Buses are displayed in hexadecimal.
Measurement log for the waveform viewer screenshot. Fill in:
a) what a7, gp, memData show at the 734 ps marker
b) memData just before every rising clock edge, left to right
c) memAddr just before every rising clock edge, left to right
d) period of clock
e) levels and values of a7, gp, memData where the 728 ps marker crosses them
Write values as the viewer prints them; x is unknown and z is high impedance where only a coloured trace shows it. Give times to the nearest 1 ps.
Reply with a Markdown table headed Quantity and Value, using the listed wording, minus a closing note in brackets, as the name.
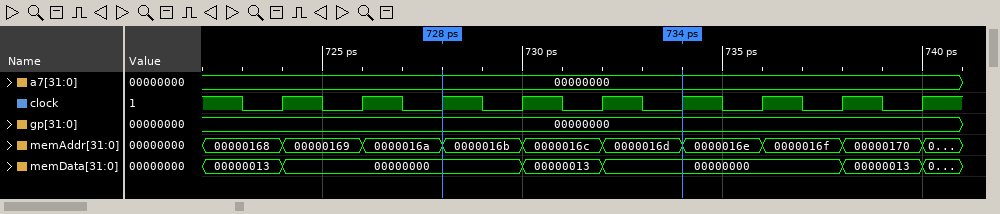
| Quantity | Value |
|---|---|
| what a7, gp, memData show at the 734 ps marker | a7=00000000, gp=00000000, memData=00000000 |
| memData just before every rising clock edge, left to right | 00000013, 00000000, 00000000, 00000000, 00000013, 00000000, 00000000, 00000000, 00000013 |
| memAddr just before every rising clock edge, left to right | 00000168, 00000169, 0000016a, 0000016b, 0000016c, 0000016d, 0000016e, 0000016f, 00000170 |
| period of clock | 2 ps |
| levels and values of a7, gp, memData where the 728 ps marker crosses them | a7=00000000, gp=00000000, memData=00000000 |
